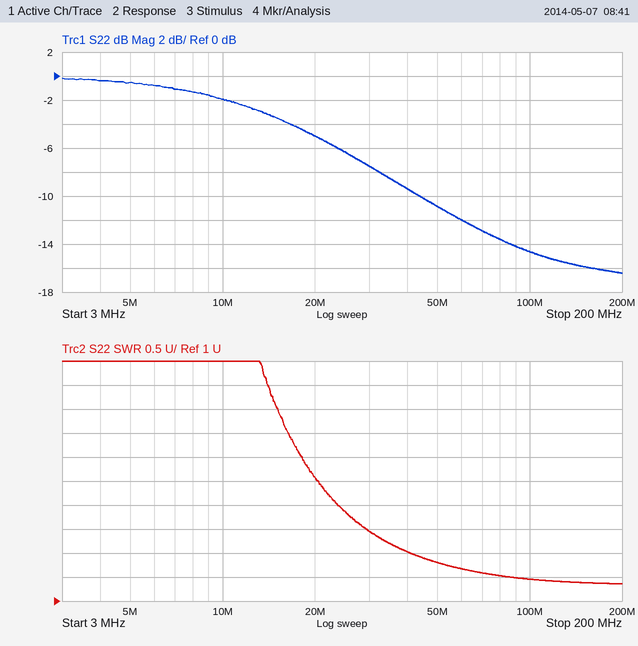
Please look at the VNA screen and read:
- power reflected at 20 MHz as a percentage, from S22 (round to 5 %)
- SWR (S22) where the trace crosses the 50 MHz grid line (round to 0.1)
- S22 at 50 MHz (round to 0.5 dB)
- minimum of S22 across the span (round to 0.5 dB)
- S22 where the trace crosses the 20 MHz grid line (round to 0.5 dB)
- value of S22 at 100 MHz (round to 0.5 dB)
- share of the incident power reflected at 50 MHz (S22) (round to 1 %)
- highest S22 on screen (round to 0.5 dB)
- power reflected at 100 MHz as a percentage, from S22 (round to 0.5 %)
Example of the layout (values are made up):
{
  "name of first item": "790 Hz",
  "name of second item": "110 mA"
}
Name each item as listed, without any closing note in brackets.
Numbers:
{
  "power reflected at 20 MHz as a percentage, from S22": "30 %",
  "SWR (S22) where the trace crosses the 50 MHz grid line": "1.8",
  "S22 at 50 MHz": "-11.0 dB",
  "minimum of S22 across the span": "-16.5 dB",
  "S22 where the trace crosses the 20 MHz grid line": "-5.0 dB",
  "value of S22 at 100 MHz": "-14.5 dB",
  "share of the incident power reflected at 50 MHz (S22)": "8 %",
  "highest S22 on screen": "0.0 dB",
  "power reflected at 100 MHz as a percentage, from S22": "3.5 %"
}
